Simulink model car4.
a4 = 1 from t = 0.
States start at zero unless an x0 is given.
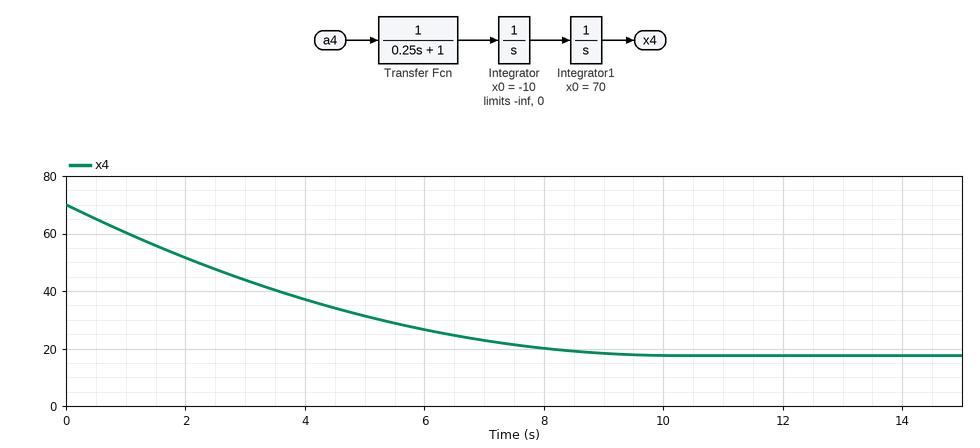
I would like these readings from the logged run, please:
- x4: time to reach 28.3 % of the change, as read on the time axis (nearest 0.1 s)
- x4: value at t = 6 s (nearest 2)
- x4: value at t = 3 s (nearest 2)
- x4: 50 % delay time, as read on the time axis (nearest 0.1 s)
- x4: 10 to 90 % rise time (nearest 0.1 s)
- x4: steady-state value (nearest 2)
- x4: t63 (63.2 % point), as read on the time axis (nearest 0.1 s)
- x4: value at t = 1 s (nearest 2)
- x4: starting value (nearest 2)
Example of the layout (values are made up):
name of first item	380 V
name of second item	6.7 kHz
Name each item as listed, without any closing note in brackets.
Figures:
x4: time to reach 28.3 % of the change, as read on the time axis	1.6 s
x4: value at t = 6 s	26
x4: value at t = 3 s	44
x4: 50 % delay time, as read on the time axis	3.0 s
x4: 10 to 90 % rise time	6.5 s
x4: steady-state value	18
x4: t63 (63.2 % point), as read on the time axis	4.0 s
x4: value at t = 1 s	60
x4: starting value	70
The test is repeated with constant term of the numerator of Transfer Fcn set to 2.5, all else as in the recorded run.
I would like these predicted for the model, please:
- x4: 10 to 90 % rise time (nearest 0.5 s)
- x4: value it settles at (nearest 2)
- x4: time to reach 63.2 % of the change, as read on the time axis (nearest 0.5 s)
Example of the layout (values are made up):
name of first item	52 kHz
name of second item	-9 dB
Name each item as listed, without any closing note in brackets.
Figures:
x4: 10 to 90 % rise time	2.5 s
x4: value it settles at	48
x4: time to reach 63.2 % of the change, as read on the time axis	1.5 s
